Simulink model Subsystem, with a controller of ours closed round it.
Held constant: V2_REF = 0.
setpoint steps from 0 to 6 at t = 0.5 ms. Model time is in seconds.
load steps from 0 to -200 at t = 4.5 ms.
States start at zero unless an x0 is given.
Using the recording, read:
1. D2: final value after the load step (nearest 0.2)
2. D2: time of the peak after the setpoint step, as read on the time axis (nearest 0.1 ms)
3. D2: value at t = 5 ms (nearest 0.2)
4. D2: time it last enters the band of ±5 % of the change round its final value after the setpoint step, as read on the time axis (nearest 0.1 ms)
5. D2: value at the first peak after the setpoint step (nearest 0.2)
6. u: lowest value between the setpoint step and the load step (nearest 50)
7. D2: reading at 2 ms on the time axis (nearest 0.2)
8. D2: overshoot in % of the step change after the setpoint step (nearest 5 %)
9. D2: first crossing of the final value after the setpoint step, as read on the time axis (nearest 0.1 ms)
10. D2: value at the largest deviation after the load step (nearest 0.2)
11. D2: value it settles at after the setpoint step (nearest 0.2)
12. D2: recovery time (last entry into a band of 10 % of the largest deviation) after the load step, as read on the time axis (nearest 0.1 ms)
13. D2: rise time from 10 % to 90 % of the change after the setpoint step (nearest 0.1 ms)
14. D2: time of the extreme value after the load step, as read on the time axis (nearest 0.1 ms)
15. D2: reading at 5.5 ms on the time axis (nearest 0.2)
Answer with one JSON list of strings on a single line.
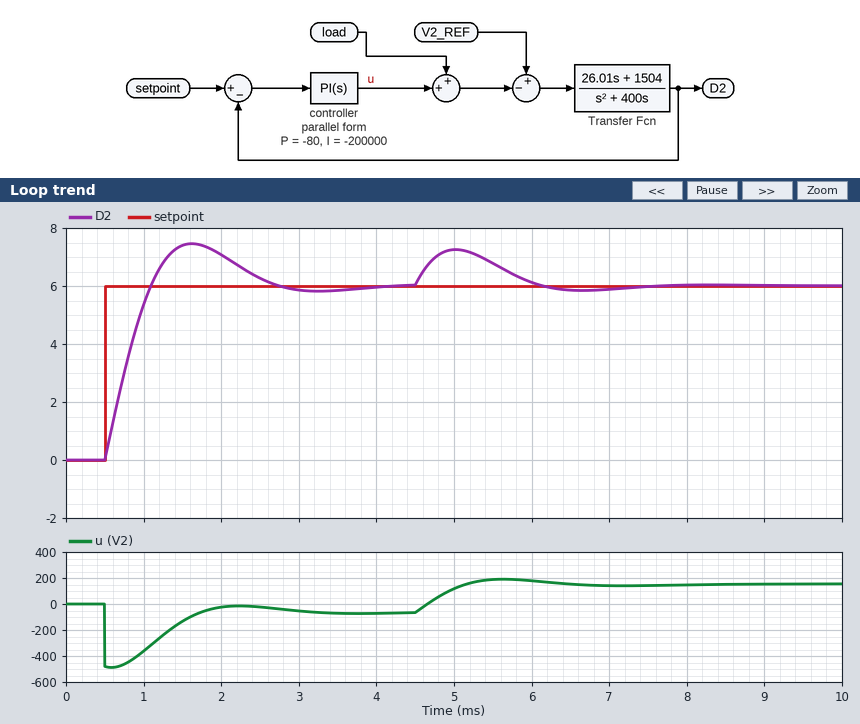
["6.0", "1.6 ms", "7.2", "2.5 ms", "7.4", "-500", "7.0", "25 %", "1.1 ms", "7.2", "6.0", "7.0 ms", "0.5 ms", "5.0 ms", "6.8"]
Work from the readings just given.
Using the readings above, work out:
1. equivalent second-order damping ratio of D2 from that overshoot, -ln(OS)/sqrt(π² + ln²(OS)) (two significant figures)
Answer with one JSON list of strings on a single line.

["0.40"]
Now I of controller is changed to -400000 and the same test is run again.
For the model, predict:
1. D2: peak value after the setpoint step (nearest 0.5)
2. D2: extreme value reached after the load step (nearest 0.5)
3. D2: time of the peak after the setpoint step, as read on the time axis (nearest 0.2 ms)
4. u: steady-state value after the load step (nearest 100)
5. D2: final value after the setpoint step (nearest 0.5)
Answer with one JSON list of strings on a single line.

["8.0", "7.0", "1.4 ms", "200", "6.0"]
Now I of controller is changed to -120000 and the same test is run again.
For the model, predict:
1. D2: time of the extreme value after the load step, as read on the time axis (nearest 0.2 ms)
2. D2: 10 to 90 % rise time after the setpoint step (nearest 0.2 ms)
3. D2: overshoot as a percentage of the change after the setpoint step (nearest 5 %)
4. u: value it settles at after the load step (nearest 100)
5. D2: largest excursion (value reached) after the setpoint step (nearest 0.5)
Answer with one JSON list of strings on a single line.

["5.2 ms", "0.6 ms", "15 %", "200", "7.0"]
